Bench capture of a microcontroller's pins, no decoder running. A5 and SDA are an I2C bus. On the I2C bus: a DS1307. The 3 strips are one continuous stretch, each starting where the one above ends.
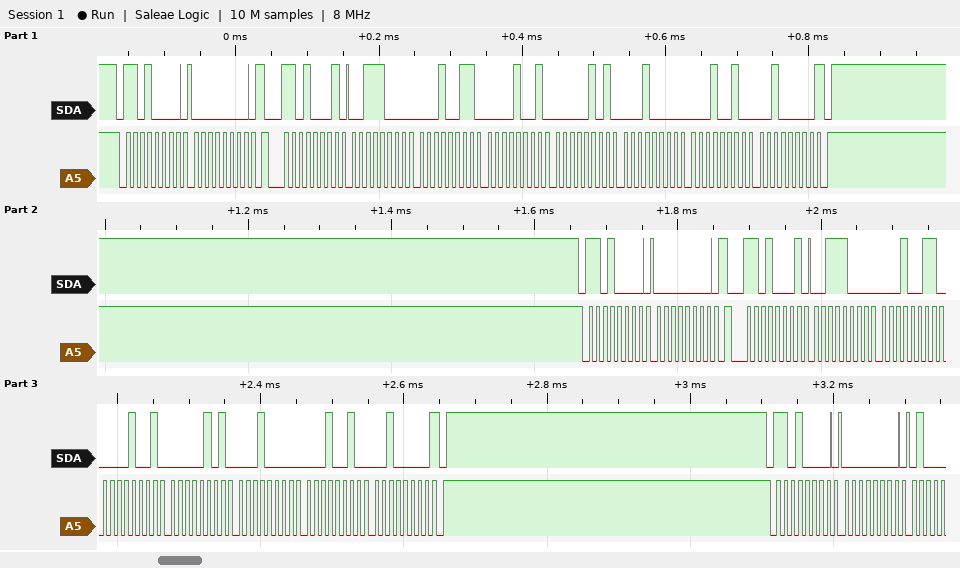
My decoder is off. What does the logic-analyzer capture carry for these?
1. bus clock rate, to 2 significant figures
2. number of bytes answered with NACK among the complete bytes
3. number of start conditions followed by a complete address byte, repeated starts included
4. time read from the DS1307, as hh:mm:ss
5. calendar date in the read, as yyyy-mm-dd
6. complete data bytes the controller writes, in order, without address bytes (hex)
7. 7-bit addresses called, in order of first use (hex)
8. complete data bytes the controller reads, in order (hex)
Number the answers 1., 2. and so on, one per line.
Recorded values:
1. 100 kHz
2. 2
3. 5
4. 09:13:38
5. 2020-12-10
6. 00 00 00
7. 0x68
8. 38 13 09 05 10 12 20 38 13 09 05 10 12 20
